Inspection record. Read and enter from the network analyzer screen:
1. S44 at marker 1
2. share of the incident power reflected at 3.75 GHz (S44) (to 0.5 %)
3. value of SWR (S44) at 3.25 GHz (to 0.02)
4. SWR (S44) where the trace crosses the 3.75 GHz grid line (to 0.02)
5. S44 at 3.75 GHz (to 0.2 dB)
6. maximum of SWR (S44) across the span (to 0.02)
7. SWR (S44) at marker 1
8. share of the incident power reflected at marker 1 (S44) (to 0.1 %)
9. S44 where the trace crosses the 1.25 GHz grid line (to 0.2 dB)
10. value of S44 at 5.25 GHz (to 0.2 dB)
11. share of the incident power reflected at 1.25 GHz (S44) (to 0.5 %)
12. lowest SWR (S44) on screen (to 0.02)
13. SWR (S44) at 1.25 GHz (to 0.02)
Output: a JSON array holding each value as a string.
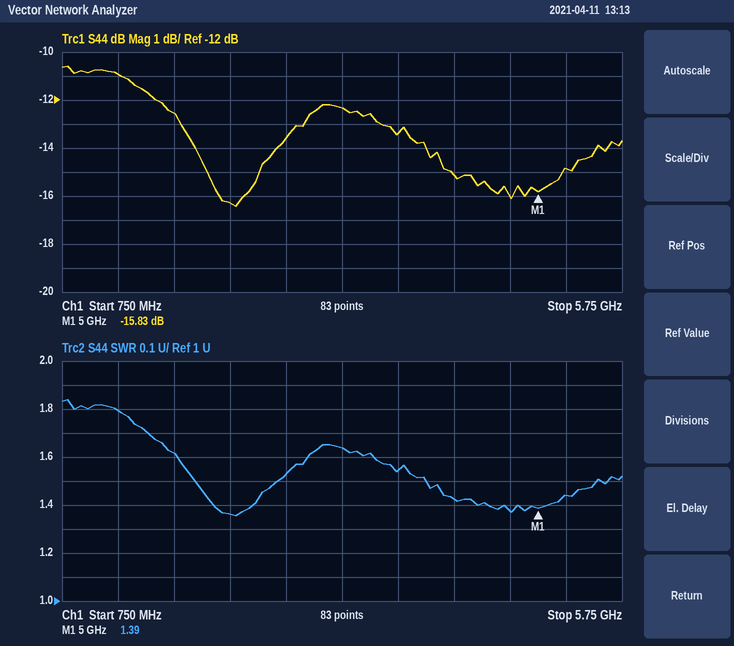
["-15.83 dB", "4.5 %", "1.64", "1.54", "-13.4 dB", "1.84", "1.39", "2.6 %", "-11.0 dB", "-14.8 dB", "8.0 %", "1.36", "1.80"]
